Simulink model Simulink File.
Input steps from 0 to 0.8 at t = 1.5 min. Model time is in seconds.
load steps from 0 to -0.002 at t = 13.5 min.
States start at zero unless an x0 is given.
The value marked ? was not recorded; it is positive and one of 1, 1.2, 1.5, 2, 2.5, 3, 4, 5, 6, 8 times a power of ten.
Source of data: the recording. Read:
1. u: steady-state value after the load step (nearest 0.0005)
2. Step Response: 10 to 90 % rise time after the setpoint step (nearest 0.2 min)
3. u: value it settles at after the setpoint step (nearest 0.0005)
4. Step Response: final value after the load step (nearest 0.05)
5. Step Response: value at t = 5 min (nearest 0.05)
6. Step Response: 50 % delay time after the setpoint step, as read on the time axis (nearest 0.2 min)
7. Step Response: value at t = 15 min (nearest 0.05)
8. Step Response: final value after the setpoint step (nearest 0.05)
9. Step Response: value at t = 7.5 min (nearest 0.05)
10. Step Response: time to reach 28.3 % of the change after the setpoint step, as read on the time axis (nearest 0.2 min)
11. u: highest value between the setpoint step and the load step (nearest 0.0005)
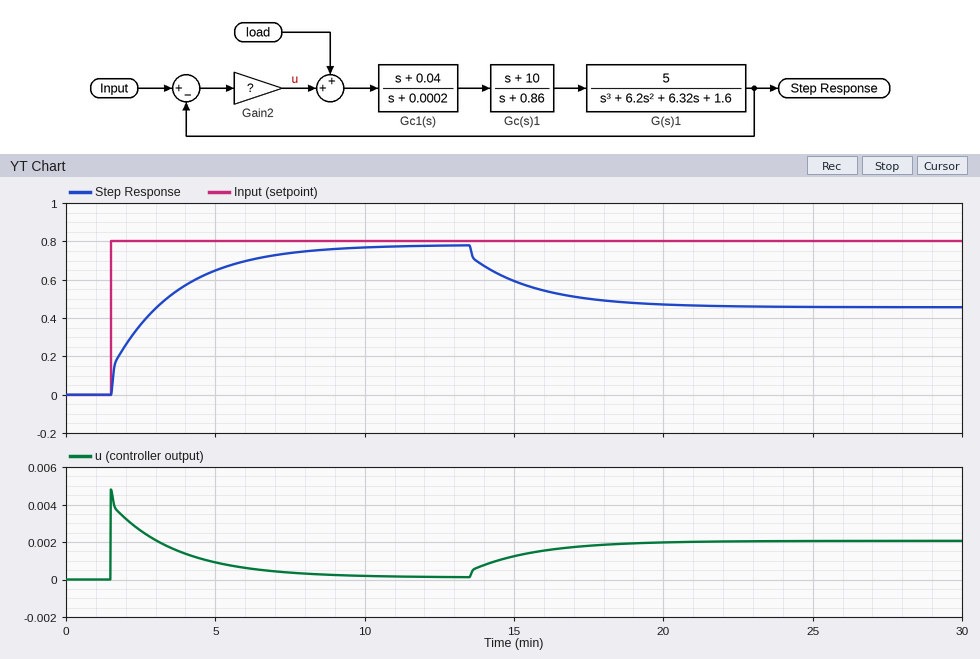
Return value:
0.0020
4.6 min
0.0000
0.45
0.65
2.6 min
0.60
0.80
0.75
1.8 min
0.0050
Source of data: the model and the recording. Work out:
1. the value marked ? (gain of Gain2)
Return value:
0.006
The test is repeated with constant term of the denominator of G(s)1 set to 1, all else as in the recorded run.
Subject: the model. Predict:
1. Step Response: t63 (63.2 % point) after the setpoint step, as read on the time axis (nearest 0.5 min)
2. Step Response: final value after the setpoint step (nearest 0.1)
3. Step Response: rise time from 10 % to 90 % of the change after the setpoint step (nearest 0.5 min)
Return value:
2.5 min
0.8
3.0 min
